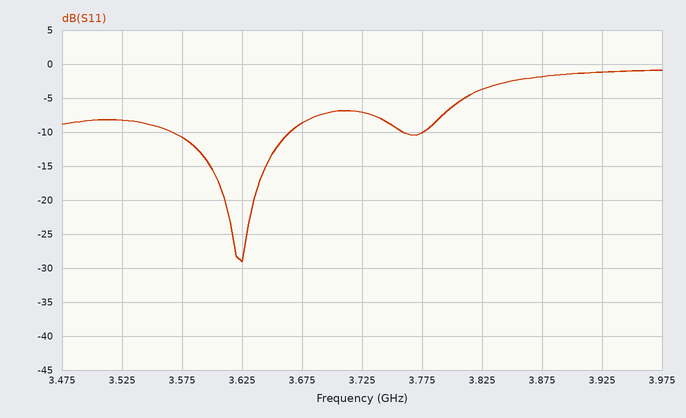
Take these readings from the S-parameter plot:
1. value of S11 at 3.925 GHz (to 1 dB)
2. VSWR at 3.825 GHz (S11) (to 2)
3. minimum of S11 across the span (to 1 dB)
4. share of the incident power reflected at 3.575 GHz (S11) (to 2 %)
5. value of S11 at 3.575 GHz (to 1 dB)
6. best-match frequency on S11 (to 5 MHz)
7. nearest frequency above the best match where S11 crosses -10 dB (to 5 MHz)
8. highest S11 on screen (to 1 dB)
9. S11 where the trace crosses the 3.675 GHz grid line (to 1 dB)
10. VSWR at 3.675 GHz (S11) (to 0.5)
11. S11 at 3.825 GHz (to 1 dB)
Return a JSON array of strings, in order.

["-1 dB", "4", "-29 dB", "8 %", "-11 dB", "3.625 GHz", "3.665 GHz", "-1 dB", "-9 dB", "2.0", "-4 dB"]
